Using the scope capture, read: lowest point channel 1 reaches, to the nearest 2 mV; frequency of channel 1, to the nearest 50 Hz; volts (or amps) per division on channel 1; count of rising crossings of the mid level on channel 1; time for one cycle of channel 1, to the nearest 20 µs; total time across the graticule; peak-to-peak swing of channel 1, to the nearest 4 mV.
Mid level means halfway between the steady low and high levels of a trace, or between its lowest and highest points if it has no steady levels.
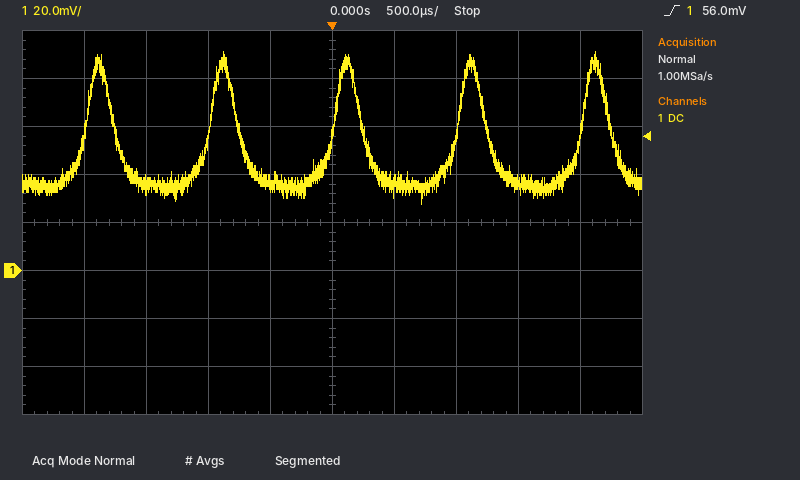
28 mV
1.00 kHz
20 mV
5
1.00 ms
5 ms
64 mV
